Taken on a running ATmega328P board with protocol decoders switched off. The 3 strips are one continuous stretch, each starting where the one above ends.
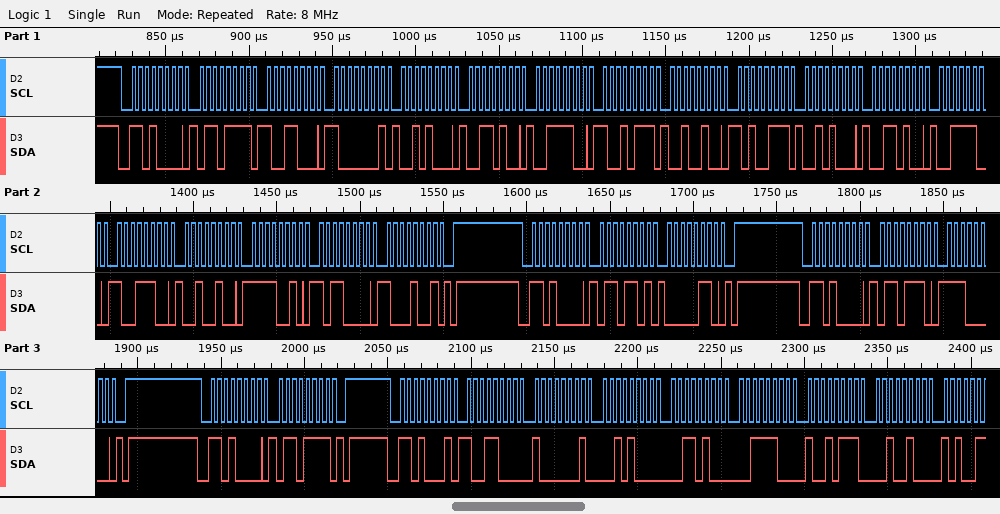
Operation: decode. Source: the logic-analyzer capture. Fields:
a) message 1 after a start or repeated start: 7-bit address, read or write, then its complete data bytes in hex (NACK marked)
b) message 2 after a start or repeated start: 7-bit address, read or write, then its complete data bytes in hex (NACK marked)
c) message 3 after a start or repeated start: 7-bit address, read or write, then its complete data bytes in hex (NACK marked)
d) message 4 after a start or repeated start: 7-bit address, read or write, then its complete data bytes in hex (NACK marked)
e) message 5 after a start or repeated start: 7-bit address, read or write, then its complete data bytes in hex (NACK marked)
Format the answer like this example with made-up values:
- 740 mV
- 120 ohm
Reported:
- 0x68 write: 6F 98 81 28 34 3C 97 24 A7 28 34 3C 9C 24 F2 B0 89
- 0x68 write: 6D 06
- 0x68 write: 6E E0
- 0x68 write: 6F
- 0x68 read: 98 81 28 34 3C 97 24
